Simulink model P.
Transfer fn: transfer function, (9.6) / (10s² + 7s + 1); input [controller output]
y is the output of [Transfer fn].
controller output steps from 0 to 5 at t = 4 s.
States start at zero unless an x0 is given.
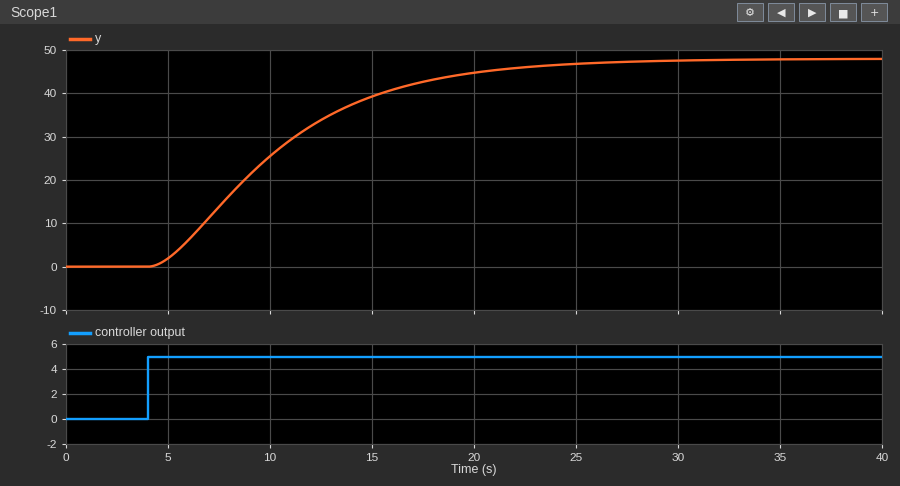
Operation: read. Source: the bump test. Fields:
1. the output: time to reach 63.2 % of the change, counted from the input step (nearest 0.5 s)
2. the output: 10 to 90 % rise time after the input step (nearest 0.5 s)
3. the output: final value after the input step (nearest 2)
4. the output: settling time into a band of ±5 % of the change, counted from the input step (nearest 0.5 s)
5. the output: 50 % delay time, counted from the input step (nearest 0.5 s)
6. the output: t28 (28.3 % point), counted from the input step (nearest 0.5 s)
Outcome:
7.5 s
12.5 s
48
17.5 s
5.5 s
3.5 s
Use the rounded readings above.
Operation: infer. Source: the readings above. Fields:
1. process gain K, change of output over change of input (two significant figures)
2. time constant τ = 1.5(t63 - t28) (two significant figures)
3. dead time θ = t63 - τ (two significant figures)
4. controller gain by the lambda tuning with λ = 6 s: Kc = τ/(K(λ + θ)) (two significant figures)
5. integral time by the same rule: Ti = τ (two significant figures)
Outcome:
9.6
6.0 s
1.5 s
0.083
6.0 s
